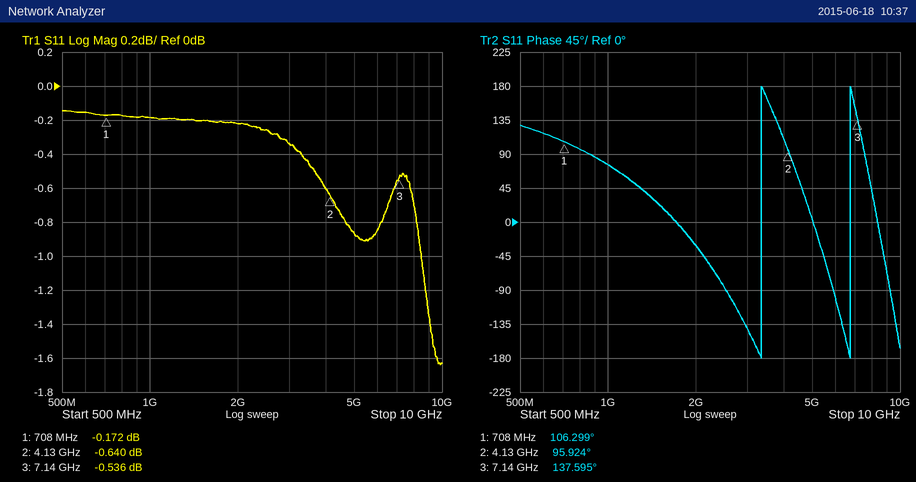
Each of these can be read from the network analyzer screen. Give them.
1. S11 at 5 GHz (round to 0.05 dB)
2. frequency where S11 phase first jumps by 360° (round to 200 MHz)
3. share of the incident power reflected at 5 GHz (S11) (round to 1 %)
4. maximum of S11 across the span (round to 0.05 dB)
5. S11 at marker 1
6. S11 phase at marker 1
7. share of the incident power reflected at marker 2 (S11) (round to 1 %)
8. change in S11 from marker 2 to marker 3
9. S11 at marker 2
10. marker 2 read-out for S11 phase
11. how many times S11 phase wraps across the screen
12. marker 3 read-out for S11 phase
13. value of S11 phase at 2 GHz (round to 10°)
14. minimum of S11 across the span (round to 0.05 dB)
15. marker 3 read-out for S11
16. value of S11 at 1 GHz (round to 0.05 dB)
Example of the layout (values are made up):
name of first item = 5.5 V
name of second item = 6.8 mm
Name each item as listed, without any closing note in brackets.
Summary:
S11 at 5 GHz = -0.85 dB
frequency where S11 phase first jumps by 360° = 3.4 GHz
share of the incident power reflected at 5 GHz (S11) = 82 %
maximum of S11 across the span = -0.15 dB
S11 at marker 1 = -0.172 dB
S11 phase at marker 1 = 106.299°
share of the incident power reflected at marker 2 (S11) = 86 %
change in S11 from marker 2 to marker 3 = 0.104 dB
S11 at marker 2 = -0.640 dB
marker 2 read-out for S11 phase = 95.924°
how many times S11 phase wraps across the screen = 2
marker 3 read-out for S11 phase = 137.595°
value of S11 phase at 2 GHz = -30°
minimum of S11 across the span = -1.65 dB
marker 3 read-out for S11 = -0.536 dB
value of S11 at 1 GHz = -0.20 dB
